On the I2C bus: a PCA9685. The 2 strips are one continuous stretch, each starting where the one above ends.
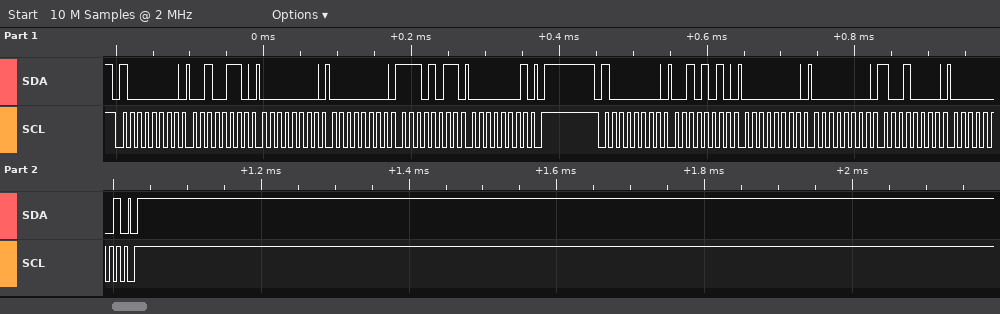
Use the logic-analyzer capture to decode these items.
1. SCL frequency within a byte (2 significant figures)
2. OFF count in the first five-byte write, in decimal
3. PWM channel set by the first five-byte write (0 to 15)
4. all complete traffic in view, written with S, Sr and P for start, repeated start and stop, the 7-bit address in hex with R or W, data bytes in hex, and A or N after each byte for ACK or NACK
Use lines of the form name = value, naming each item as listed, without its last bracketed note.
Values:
SCL frequency within a byte = 100 kHz
OFF count in the first five-byte write, in decimal = 491
PWM channel set by the first five-byte write = 8
all complete traffic in view, written with S, Sr and P for start, repeated start and stop, the 7-bit address in hex with R or W, data bytes in hex, and A or N after each byte for ACK or NACK = S 40W A 26 A 00 A 00 A EB A 01 A P S 40W A 2A A 00 A 00 A 90 A 01 A P
